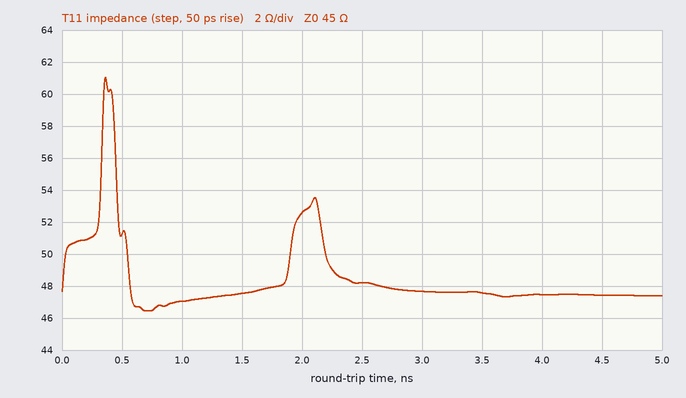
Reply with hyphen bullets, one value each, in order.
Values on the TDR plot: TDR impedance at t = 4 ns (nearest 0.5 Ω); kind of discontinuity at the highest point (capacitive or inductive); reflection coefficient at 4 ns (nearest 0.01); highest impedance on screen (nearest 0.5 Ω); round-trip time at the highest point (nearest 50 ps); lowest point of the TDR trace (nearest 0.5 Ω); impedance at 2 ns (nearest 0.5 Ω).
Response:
- 47.5 Ω
- inductive
- +0.03
- 61.0 Ω
- 350 ps
- 46.5 Ω
- 52.5 Ω
